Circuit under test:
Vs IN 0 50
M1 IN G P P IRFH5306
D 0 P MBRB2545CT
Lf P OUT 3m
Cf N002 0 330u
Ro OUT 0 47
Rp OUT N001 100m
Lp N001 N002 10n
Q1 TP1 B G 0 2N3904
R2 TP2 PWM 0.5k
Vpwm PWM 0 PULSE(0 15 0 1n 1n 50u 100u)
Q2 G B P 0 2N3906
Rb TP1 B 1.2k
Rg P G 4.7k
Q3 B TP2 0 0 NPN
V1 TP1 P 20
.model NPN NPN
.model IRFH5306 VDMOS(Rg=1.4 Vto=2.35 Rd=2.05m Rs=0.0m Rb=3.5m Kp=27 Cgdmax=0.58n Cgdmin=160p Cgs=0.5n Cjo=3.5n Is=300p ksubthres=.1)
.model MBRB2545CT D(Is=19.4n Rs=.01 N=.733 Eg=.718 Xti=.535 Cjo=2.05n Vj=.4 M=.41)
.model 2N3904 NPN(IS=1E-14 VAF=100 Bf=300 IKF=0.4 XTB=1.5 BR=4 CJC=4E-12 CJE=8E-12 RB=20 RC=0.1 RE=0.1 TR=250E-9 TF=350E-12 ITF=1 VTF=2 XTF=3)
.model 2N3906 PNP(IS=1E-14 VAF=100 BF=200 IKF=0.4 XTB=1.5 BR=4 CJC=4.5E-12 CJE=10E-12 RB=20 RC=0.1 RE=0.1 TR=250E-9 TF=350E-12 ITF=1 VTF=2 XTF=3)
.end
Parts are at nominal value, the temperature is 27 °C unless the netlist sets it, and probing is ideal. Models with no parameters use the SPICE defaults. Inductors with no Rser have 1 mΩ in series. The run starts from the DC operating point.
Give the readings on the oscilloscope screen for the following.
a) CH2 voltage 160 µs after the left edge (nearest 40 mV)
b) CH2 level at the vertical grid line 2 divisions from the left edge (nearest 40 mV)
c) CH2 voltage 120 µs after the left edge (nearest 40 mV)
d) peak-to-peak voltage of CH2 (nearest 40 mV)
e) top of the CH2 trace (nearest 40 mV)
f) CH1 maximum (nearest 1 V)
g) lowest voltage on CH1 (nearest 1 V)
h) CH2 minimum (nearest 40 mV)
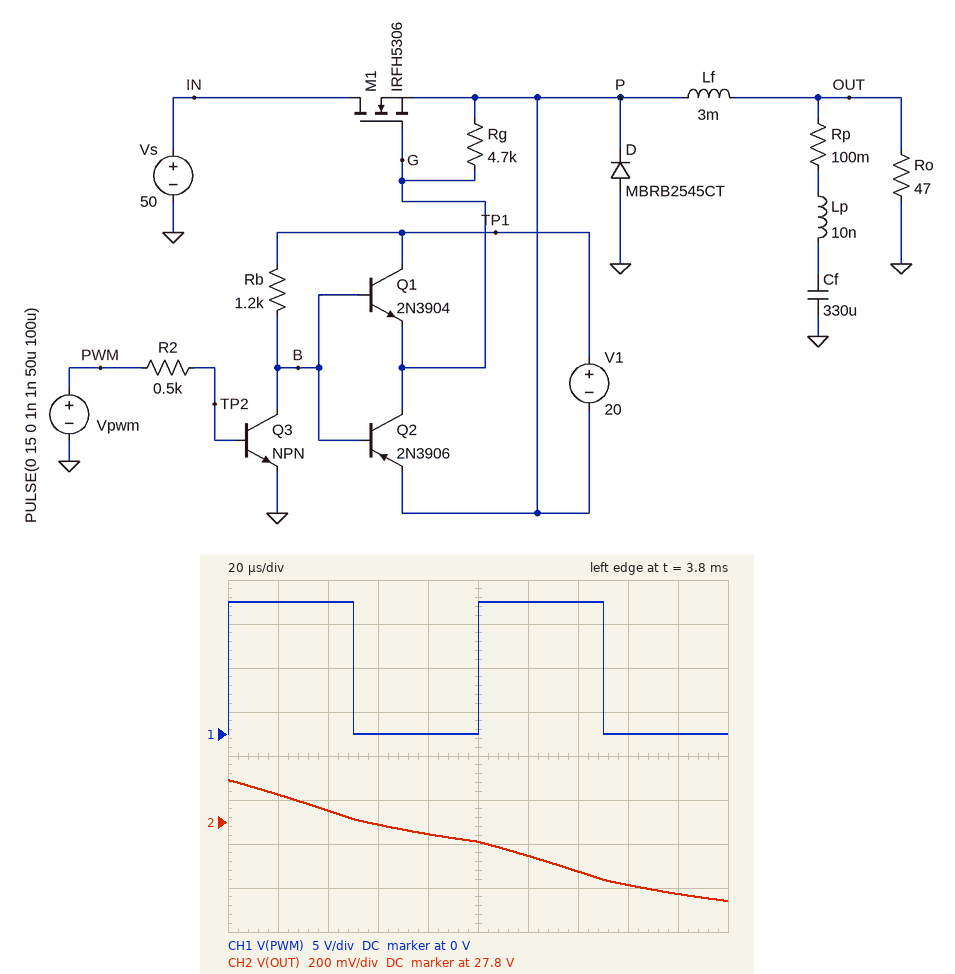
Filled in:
27.52 V
27.84 V
27.64 V
560 mV
28.00 V
15 V
0 V
27.44 V
